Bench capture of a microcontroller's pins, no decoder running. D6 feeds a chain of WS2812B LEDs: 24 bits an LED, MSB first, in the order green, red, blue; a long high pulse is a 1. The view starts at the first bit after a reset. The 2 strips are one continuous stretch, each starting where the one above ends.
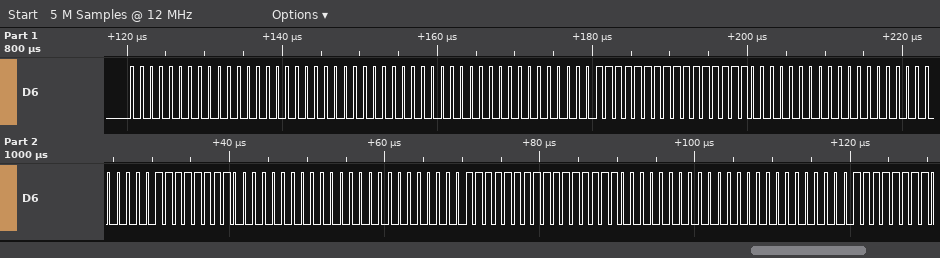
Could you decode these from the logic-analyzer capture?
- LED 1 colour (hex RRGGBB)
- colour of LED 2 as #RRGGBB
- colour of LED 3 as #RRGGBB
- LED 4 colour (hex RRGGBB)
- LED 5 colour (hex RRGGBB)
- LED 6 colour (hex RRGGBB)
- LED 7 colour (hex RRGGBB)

#000000
#000000
#FFFF00
#0000FF
#000000
#FFFF00
#0000FF
